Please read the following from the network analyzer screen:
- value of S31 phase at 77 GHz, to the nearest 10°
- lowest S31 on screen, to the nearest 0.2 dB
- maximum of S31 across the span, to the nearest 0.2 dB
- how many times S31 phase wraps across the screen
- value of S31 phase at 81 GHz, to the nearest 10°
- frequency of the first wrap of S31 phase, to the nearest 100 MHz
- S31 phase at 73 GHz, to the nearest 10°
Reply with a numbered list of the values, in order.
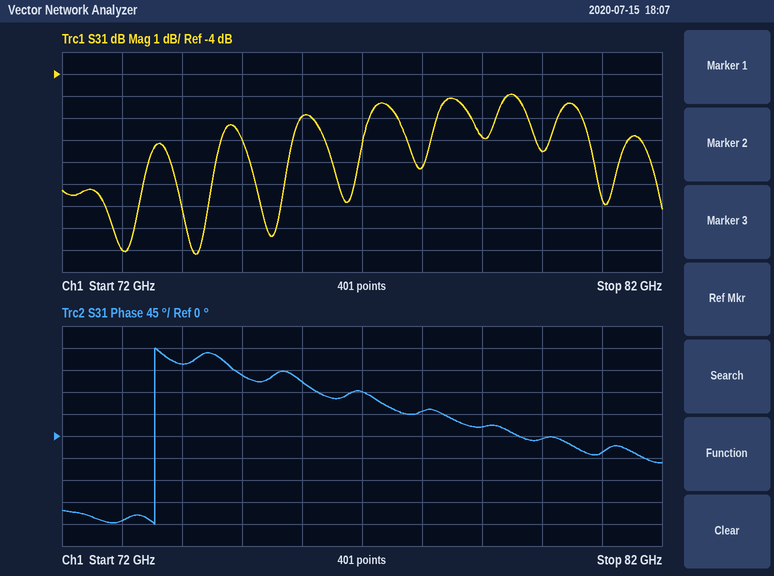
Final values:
1. 90°
2. -12.2 dB
3. -5.0 dB
4. 1
5. -30°
6. 73.5 GHz
7. -170°
